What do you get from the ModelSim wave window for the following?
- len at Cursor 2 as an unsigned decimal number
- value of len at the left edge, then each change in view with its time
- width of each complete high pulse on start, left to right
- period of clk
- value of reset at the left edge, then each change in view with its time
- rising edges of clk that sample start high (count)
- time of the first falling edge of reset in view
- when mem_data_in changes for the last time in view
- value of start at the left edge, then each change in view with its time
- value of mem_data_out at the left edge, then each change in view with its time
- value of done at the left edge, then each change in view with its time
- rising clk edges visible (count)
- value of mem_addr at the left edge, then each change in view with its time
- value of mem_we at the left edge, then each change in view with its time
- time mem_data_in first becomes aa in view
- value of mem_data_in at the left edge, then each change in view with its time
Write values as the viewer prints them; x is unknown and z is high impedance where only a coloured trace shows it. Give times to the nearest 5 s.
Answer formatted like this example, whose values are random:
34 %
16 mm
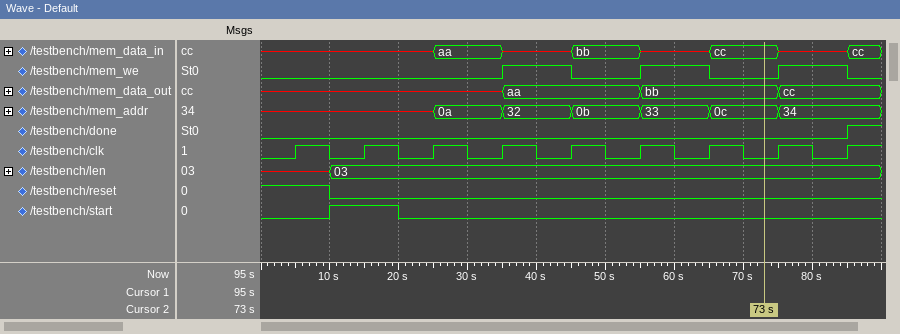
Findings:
3
x, 03 at 10 s
10 s
10 s
1, 0 at 10 s
1
10 s
85 s
0, 1 at 10 s, 0 at 20 s
x, aa at 35 s, bb at 55 s, cc at 75 s
0, 1 at 85 s
9
x, 0a at 25 s, 32 at 35 s, 0b at 45 s, 33 at 55 s, 0c at 65 s, 34 at 75 s
0, 1 at 35 s, 0 at 45 s, 1 at 55 s, 0 at 65 s, 1 at 75 s, 0 at 85 s
25 s
x, aa at 25 s, x at 35 s, bb at 45 s, x at 55 s, cc at 65 s, x at 75 s, cc at 85 s
